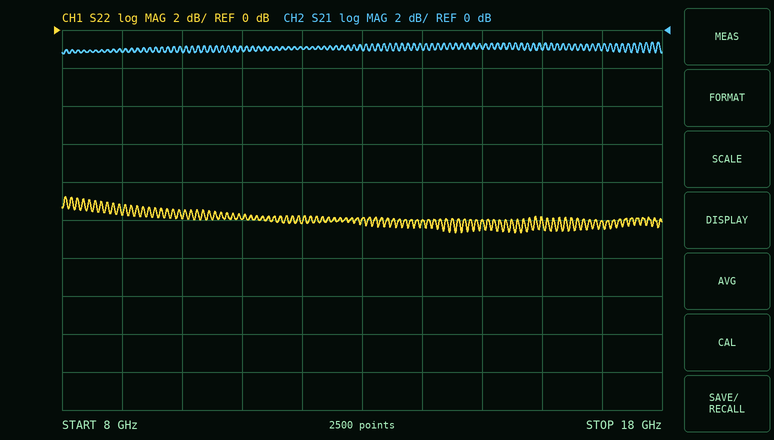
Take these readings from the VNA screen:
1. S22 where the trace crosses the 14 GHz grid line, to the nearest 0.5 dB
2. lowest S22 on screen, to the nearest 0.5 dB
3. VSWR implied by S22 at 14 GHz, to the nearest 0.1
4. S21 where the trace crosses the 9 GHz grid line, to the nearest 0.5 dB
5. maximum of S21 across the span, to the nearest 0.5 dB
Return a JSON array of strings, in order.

["-10.0 dB", "-10.5 dB", "1.9", "-1.0 dB", "-0.5 dB"]
